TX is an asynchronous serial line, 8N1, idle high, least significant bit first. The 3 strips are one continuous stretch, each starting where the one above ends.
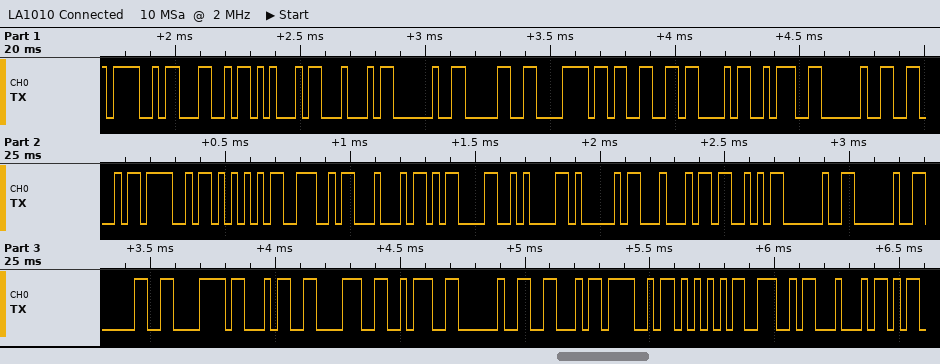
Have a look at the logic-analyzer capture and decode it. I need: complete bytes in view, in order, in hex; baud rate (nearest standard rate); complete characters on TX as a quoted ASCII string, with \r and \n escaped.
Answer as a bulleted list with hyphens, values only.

- 4F 4C 45 44 20 30 78 33 43 3A 20 46 4F 55 4E 44 0D 0A 41 44 53 20 20 30 78 34 38 3A 20 46 4F 55 4E 44
- 38400 baud
- "OLED 0x3C: FOUND\r\nADS  0x48: FOUND"
